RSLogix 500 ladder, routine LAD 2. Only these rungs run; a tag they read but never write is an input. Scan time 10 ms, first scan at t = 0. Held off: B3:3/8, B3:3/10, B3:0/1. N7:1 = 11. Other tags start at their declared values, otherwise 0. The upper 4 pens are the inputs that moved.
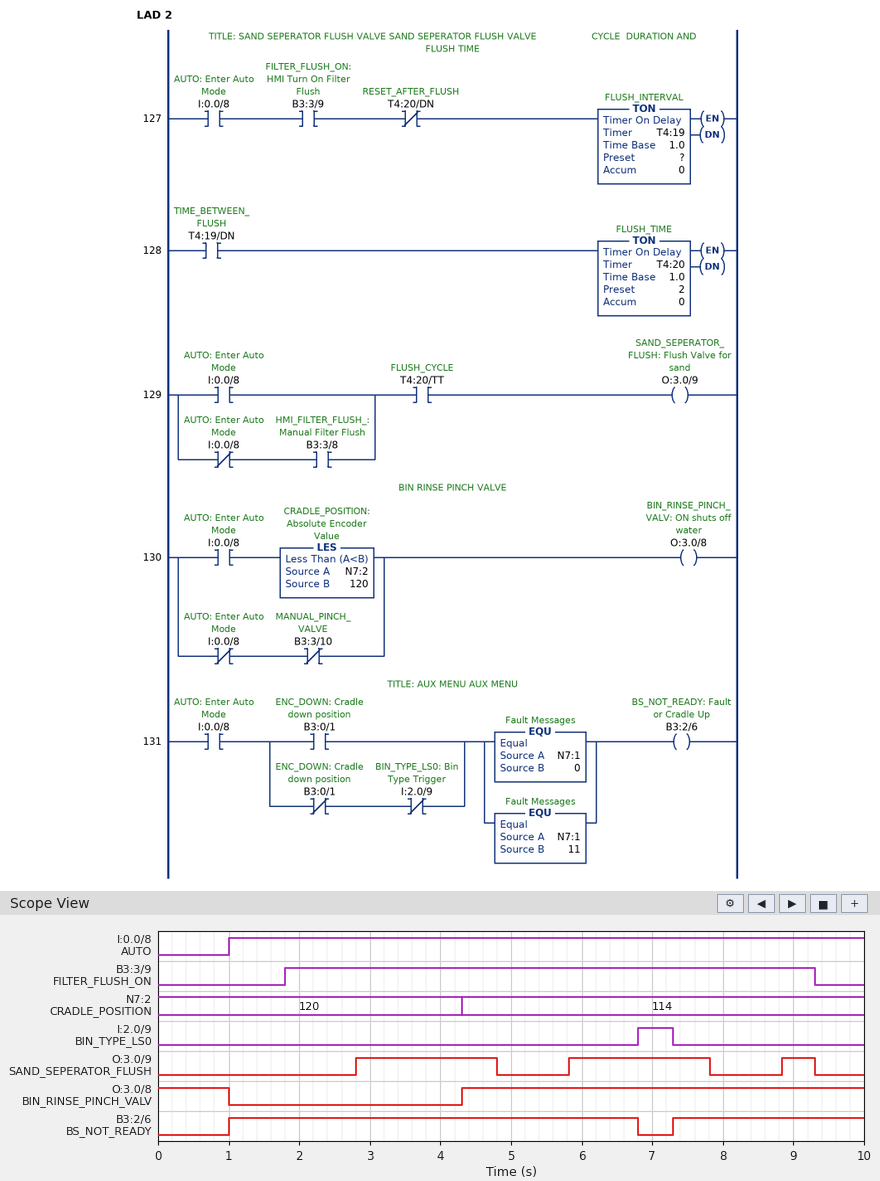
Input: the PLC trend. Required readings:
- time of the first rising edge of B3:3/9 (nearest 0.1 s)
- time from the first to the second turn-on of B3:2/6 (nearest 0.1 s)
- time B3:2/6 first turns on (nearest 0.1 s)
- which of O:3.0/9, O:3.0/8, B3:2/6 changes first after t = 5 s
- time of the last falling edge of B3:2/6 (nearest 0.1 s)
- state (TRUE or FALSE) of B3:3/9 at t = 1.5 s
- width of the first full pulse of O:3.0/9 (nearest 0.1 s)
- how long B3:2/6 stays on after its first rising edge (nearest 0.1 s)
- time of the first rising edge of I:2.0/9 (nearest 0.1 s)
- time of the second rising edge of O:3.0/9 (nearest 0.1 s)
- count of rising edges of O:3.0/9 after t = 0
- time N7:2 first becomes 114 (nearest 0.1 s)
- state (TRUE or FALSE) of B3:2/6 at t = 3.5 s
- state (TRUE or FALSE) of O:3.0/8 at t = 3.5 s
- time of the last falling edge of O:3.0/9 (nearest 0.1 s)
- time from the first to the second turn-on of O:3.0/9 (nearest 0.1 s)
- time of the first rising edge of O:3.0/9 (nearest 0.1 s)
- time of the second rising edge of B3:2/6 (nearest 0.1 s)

1.8 s
6.3 s
1.0 s
O:3.0/9
6.8 s
FALSE
2.0 s
5.8 s
6.8 s
5.8 s
3
4.3 s
TRUE
FALSE
9.3 s
3.0 s
2.8 s
7.3 s
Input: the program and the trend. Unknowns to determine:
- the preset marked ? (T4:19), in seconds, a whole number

1 s
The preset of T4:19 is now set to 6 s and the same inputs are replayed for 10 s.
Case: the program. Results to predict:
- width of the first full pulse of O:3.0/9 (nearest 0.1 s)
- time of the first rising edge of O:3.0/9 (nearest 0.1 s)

1.5 s
7.8 s
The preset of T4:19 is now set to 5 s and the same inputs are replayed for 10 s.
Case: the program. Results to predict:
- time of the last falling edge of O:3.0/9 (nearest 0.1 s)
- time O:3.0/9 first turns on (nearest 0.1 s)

8.8 s
6.8 s
